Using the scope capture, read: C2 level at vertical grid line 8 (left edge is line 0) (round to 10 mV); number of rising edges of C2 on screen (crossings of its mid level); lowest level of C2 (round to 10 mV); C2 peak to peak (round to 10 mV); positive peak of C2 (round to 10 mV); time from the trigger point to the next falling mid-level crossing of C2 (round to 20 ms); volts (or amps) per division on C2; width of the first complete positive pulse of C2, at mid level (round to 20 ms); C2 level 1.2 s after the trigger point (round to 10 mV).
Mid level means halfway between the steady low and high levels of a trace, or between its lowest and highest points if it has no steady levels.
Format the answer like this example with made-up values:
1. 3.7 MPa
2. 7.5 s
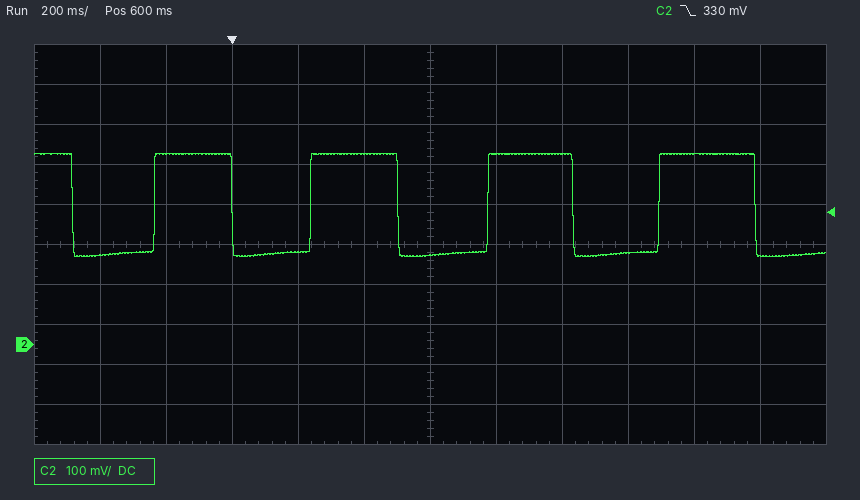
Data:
1. 480 mV
2. 4
3. 220 mV
4. 260 mV
5. 480 mV
6. 500 ms
7. 100 mV
8. 240 ms
9. 230 mV
